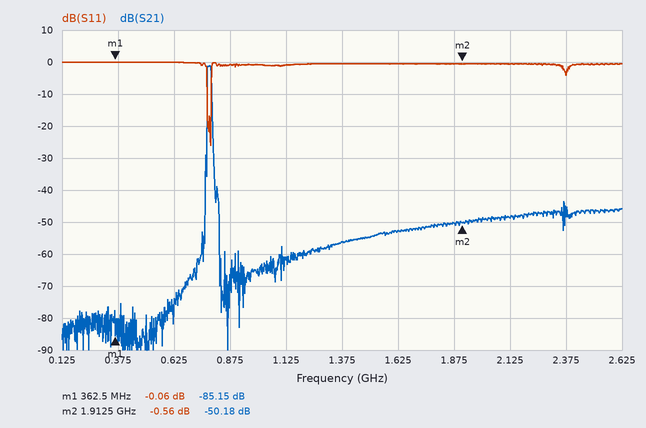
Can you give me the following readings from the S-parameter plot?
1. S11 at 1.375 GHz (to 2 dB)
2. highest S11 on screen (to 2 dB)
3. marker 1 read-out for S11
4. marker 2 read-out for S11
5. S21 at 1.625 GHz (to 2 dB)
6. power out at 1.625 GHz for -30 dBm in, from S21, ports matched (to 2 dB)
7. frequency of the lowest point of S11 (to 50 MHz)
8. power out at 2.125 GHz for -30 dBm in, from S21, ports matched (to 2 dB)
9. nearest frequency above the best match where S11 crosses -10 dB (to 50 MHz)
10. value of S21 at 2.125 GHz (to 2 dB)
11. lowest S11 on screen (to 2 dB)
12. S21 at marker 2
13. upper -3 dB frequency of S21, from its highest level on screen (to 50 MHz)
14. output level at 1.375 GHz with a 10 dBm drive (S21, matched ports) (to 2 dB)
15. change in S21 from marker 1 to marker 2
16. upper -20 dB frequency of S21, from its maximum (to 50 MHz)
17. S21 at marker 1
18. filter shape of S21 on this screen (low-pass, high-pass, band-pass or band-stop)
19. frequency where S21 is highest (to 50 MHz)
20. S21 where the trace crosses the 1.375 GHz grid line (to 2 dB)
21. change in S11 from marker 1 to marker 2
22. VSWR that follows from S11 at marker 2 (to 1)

0 dB
0 dB
-0.06 dB
-0.56 dB
-52 dB
-82 dBm
800 MHz
-78 dBm
800 MHz
-48 dB
-26 dB
-50.18 dB
800 MHz
-46 dBm
34.97 dB
800 MHz
-85.15 dB
band-pass
800 MHz
-56 dB
-0.50 dB
31
